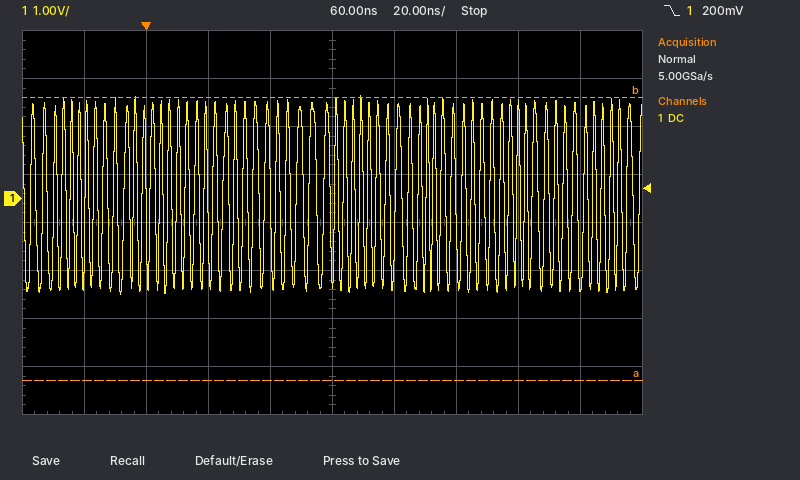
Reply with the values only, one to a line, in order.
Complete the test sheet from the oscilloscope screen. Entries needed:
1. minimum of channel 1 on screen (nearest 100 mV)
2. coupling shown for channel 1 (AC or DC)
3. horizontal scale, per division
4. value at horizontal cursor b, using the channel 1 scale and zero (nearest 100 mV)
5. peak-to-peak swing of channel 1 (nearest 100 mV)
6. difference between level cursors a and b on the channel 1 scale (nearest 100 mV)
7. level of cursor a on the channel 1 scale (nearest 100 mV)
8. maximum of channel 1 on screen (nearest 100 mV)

-2.0 V
DC
20 ns
2.1 V
4.1 V
5.9 V
-3.8 V
2.1 V
